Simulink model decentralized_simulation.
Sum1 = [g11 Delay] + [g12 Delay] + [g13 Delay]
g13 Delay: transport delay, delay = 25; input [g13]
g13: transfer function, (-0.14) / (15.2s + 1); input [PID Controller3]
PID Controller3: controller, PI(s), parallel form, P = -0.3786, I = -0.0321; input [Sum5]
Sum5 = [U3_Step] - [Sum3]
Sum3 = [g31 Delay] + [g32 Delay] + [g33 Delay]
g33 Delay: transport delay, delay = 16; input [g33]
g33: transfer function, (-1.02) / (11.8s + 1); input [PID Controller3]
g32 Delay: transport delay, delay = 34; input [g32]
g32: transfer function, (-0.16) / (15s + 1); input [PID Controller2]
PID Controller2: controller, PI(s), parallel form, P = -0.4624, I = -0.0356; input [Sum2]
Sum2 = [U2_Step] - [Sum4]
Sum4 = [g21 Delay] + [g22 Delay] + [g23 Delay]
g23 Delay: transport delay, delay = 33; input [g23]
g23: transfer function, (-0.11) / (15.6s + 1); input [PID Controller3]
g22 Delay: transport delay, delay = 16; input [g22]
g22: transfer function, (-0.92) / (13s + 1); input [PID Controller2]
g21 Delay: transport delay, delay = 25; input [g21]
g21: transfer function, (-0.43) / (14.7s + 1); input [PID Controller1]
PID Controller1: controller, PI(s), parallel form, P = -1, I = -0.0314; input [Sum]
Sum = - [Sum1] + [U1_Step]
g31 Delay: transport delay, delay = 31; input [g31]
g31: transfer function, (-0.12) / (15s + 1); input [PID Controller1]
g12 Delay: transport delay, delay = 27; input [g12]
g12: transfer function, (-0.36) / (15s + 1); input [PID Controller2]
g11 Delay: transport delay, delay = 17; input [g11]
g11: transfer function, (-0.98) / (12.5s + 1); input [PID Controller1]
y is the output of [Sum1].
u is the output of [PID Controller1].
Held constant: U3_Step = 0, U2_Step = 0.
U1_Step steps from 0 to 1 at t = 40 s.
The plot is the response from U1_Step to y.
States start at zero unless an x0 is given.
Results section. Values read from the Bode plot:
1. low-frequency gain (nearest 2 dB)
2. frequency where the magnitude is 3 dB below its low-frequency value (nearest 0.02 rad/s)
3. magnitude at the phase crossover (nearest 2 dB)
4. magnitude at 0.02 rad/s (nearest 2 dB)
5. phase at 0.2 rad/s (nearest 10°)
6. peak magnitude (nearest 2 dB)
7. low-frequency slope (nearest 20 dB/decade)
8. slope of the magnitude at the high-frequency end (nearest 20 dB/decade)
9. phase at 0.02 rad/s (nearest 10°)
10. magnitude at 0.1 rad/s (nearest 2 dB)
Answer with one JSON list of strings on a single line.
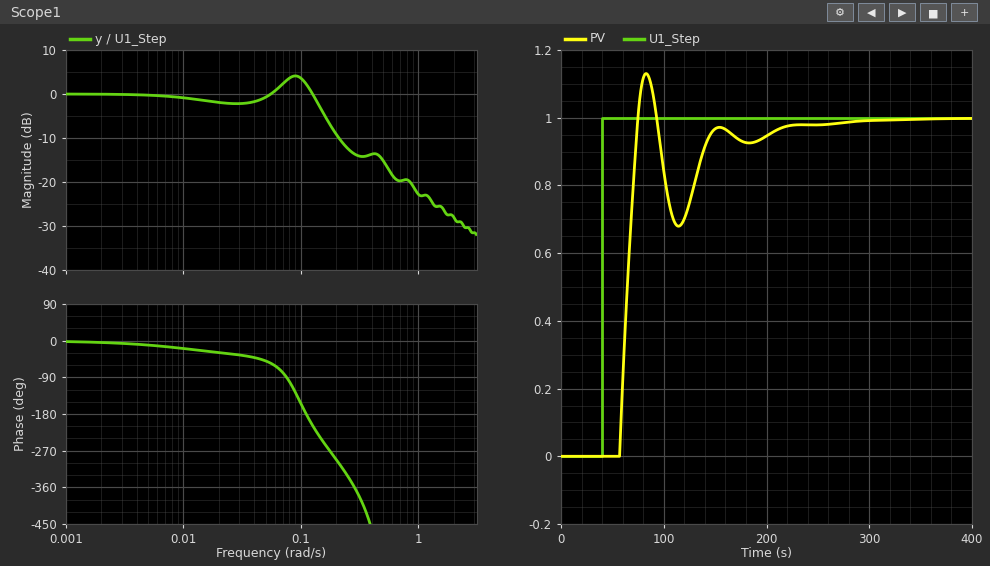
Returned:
["0 dB", "0.14 rad/s", "2 dB", "-2 dB", "-290°", "4 dB", "0 dB/decade", "-20 dB/decade", "-30°", "4 dB"]
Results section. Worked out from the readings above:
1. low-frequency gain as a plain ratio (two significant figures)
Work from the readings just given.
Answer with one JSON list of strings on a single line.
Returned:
["1.0"]
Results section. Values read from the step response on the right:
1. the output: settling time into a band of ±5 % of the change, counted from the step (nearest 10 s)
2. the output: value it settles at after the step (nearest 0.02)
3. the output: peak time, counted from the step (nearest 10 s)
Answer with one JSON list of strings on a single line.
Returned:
["160 s", "1.00", "40 s"]
